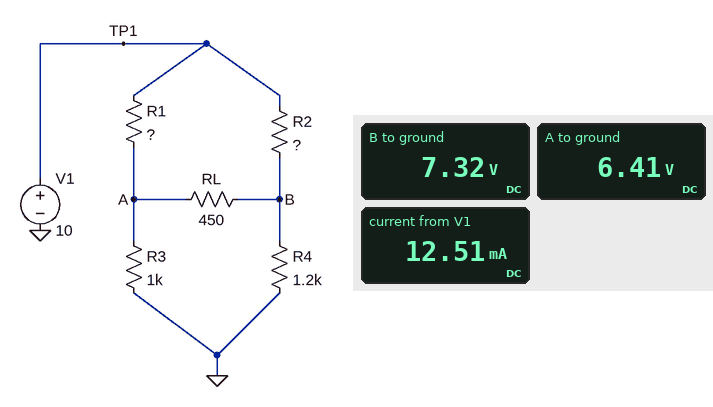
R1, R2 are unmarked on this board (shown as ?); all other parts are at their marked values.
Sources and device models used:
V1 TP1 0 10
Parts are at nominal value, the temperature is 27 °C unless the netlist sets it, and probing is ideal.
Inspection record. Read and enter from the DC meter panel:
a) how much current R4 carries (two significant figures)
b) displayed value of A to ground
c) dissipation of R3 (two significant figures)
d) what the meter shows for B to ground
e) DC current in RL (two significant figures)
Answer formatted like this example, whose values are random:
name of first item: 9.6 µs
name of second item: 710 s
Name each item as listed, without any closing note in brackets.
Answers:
how much current R4 carries: 6.1 mA
displayed value of A to ground: 6.41 V
dissipation of R3: 41 mW
what the meter shows for B to ground: 7.32 V
DC current in RL: 2.0 mA
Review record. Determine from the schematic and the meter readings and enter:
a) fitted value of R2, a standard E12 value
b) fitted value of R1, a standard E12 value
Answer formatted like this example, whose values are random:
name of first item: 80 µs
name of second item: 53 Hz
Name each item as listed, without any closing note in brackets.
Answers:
fitted value of R2, a standard E12 value: 330 Ω
fitted value of R1, a standard E12 value: 820 Ω
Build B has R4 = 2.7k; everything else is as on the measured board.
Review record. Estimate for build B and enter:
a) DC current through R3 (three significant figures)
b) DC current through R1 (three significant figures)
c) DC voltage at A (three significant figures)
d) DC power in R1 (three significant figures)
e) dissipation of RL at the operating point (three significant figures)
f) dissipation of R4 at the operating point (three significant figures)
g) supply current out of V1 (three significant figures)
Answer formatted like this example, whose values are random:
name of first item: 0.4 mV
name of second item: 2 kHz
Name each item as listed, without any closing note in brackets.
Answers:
DC current through R3: 6.78 mA
DC current through R1: 3.92 mA
DC voltage at A: 6.78 V
DC power in R1: 12.6 mW
dissipation of RL at the operating point: 3.68 mW
dissipation of R4 at the operating point: 24.1 mW
supply current out of V1: 9.77 mA
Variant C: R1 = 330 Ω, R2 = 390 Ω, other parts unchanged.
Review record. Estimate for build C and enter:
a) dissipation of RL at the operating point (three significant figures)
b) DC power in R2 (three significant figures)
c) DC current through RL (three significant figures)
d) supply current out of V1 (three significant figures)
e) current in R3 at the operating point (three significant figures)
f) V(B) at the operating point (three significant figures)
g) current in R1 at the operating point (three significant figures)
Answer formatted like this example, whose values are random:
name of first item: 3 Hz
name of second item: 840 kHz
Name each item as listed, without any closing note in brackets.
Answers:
dissipation of RL at the operating point: 368 nW
DC power in R2: 15.5 mW
DC current through RL: 28.6 µA
supply current out of V1: 13.8 mA
current in R3 at the operating point: 7.53 mA
V(B) at the operating point: 7.54 V
current in R1 at the operating point: 7.50 mA
